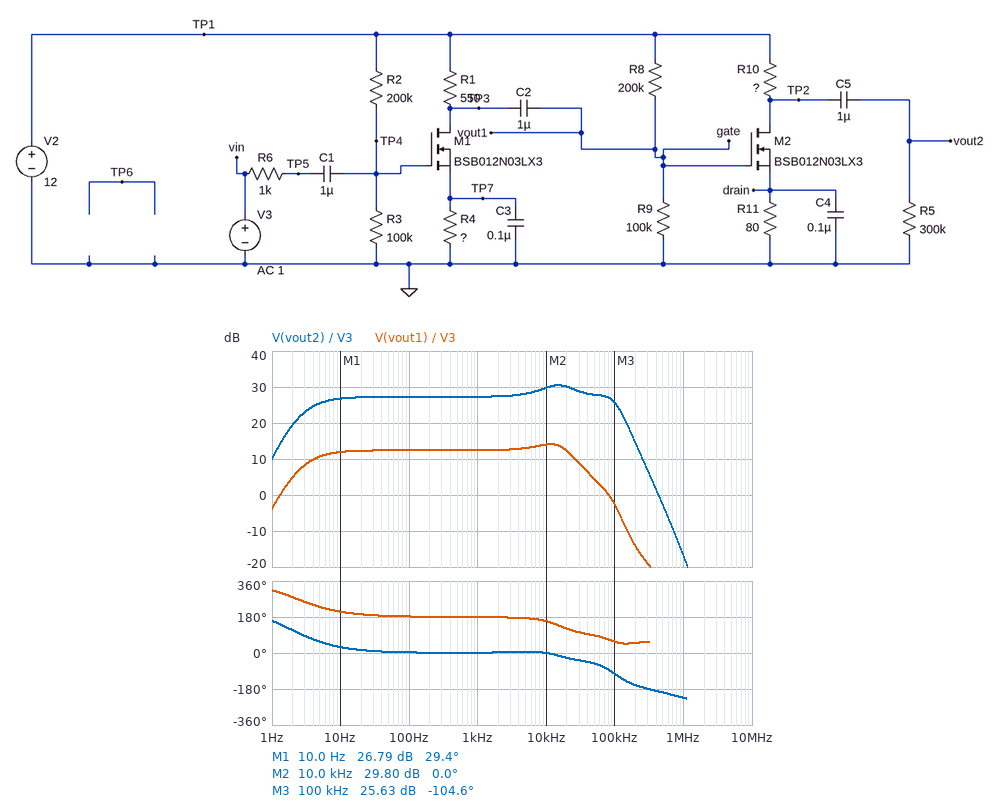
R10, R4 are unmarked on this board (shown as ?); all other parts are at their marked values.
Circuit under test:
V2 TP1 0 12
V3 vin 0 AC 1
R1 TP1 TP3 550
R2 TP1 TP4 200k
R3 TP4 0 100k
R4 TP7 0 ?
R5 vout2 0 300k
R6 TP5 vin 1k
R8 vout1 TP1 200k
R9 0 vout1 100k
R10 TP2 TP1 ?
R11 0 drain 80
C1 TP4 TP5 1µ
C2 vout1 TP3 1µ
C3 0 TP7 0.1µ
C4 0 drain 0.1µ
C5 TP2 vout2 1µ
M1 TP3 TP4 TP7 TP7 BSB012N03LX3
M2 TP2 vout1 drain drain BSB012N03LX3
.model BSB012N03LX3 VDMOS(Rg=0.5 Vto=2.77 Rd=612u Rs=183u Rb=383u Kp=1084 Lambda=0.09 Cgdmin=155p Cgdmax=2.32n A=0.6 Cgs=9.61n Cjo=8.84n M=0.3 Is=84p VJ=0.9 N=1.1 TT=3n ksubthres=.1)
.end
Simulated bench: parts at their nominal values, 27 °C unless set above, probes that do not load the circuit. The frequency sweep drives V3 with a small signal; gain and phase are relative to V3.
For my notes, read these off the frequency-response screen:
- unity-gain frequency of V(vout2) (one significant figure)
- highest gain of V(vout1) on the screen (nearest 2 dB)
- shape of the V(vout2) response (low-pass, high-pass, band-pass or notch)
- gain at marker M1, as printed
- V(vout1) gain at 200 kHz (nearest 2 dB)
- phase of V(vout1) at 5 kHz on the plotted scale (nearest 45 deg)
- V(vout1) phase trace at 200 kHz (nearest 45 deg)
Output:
400 kHz
14 dB
band-pass
26.79 dB
-14 dB
180 deg
45 deg
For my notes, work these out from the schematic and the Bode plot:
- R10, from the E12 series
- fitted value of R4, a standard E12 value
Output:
470 Ω
120 Ω
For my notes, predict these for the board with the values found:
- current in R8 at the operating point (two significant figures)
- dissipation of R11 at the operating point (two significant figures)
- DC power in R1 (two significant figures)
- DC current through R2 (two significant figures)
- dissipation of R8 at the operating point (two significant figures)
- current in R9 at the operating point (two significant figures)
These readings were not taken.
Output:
40 µA
29 mW
91 mW
40 µA
320 µW
40 µA
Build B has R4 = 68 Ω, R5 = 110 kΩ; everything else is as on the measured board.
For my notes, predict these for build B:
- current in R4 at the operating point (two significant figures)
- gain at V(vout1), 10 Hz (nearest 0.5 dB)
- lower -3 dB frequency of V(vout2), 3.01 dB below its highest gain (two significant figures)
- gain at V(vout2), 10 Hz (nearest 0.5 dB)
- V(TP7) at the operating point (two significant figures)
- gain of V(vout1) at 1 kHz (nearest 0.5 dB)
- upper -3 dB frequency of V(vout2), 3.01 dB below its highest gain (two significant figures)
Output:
19 mA
-48.5 dB
14 kHz
-34.0 dB
1.3 V
-45.0 dB
110 kHz
